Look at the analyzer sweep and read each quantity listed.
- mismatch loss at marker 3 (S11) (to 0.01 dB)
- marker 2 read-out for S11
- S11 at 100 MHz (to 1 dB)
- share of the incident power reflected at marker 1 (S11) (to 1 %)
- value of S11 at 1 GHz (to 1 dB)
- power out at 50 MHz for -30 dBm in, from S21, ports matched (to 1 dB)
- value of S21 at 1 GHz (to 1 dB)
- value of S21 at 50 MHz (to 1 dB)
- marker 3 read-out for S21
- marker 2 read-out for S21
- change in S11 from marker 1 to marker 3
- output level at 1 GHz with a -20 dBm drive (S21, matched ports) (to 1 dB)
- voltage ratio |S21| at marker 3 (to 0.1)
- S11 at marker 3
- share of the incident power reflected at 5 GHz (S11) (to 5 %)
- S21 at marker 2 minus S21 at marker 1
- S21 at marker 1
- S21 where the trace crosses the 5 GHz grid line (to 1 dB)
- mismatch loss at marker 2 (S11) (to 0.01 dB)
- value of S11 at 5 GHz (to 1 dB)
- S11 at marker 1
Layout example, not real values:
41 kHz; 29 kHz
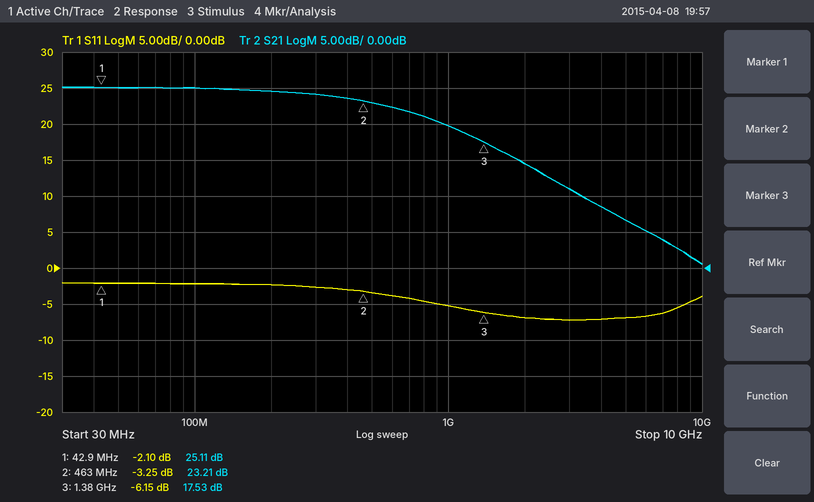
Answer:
1.21 dB; -3.25 dB; -2 dB; 62 %; -5 dB; -5 dBm; 20 dB; 25 dB; 17.53 dB; 23.21 dB; -4.05 dB; 0 dBm; 7.5; -6.15 dB; 20 %; -1.90 dB; 25.11 dB; 7 dB; 2.78 dB; -7 dB; -2.10 dB
